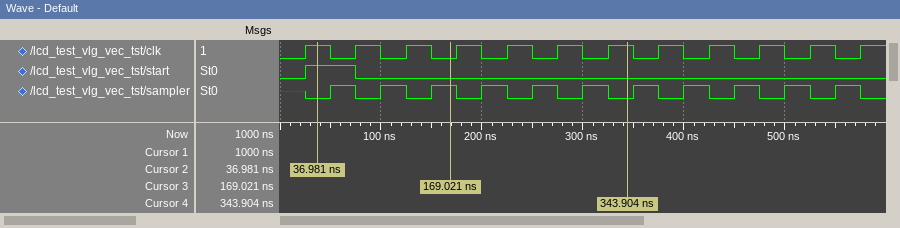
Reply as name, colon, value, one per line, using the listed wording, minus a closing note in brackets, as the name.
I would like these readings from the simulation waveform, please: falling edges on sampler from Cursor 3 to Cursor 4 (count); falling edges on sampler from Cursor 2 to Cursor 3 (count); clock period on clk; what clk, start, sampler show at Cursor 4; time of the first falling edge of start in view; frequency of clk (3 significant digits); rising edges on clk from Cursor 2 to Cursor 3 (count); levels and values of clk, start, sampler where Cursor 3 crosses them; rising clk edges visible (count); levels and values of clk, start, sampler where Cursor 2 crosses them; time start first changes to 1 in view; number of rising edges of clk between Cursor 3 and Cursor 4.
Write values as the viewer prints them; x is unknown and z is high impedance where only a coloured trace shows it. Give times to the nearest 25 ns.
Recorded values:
falling edges on sampler from Cursor 3 to Cursor 4: 4
falling edges on sampler from Cursor 2 to Cursor 3: 2
clock period on clk: 50 ns
what clk, start, sampler show at Cursor 4: clk=1, start=0, sampler=0
time of the first falling edge of start in view: 75 ns
frequency of clk: 20.0 MHz
rising edges on clk from Cursor 2 to Cursor 3: 2
levels and values of clk, start, sampler where Cursor 3 crosses them: clk=0, start=0, sampler=1
rising clk edges visible: 12
levels and values of clk, start, sampler where Cursor 2 crosses them: clk=1, start=1, sampler=0
time start first changes to 1 in view: 25 ns
number of rising edges of clk between Cursor 3 and Cursor 4: 4
